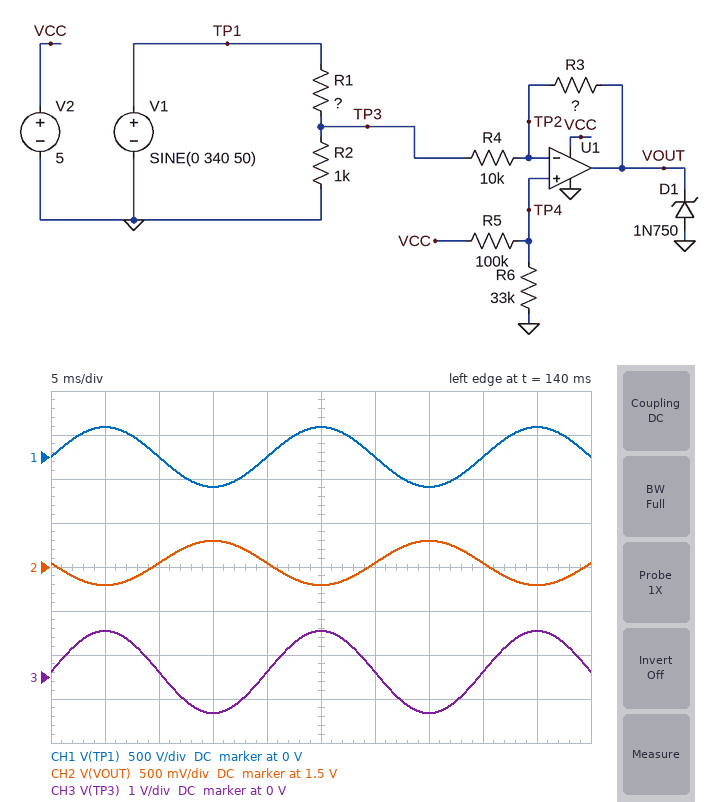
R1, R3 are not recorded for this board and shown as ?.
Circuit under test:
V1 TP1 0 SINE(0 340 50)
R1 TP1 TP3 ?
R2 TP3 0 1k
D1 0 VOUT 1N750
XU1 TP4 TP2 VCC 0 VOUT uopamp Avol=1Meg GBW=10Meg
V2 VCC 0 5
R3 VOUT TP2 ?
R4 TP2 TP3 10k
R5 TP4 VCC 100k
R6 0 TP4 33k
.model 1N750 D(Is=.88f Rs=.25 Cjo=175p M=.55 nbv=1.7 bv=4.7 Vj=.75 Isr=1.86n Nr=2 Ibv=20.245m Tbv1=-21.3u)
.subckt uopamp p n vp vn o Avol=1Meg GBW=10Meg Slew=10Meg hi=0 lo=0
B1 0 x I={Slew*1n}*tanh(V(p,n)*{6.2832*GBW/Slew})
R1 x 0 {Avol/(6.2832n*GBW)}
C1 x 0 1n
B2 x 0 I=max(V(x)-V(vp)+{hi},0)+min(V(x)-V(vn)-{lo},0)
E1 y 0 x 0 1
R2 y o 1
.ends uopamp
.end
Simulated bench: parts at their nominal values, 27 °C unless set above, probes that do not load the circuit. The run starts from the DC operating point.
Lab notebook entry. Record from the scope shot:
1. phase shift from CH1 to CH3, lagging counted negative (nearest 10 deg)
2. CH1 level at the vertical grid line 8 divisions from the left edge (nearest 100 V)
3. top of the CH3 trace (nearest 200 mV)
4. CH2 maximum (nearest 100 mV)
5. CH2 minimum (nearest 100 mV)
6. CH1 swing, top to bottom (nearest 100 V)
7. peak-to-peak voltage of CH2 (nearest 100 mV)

0 deg
0 V
1.0 V
1.8 V
1.3 V
700 V
500 mV
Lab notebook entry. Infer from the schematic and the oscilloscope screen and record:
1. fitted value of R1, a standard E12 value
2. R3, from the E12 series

330 kΩ
2.7 kΩ
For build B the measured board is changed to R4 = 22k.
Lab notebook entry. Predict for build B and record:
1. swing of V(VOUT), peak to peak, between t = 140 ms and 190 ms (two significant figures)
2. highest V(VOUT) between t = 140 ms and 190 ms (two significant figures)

240 mV
1.5 V
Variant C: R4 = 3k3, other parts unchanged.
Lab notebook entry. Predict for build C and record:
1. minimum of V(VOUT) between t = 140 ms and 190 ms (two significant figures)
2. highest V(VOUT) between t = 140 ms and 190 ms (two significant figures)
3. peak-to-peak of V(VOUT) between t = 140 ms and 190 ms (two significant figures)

1.4 V
2.7 V
1.3 V
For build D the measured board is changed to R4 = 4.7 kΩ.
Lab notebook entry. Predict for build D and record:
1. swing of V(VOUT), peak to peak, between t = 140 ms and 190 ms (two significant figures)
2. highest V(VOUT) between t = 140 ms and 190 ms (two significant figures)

970 mV
2.3 V
